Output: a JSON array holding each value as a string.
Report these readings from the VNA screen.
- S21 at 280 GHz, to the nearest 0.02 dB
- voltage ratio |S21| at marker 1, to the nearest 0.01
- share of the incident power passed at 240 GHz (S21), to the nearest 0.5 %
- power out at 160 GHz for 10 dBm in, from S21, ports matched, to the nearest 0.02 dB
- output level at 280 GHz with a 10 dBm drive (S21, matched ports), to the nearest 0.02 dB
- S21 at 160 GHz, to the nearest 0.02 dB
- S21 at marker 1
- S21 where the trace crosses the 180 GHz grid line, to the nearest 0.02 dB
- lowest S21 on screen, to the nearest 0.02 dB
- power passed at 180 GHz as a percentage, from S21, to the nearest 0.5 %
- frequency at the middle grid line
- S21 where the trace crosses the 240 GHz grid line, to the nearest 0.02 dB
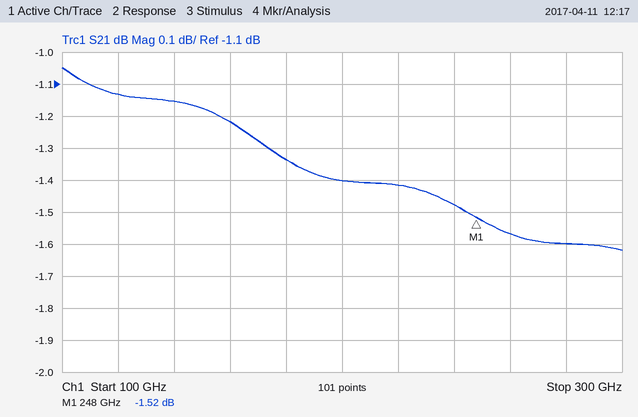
["-1.60 dB", "0.84", "71.0 %", "8.78 dBm", "8.40 dBm", "-1.22 dB", "-1.52 dB", "-1.34 dB", "-1.62 dB", "73.5 %", "200 GHz", "-1.48 dB"]
